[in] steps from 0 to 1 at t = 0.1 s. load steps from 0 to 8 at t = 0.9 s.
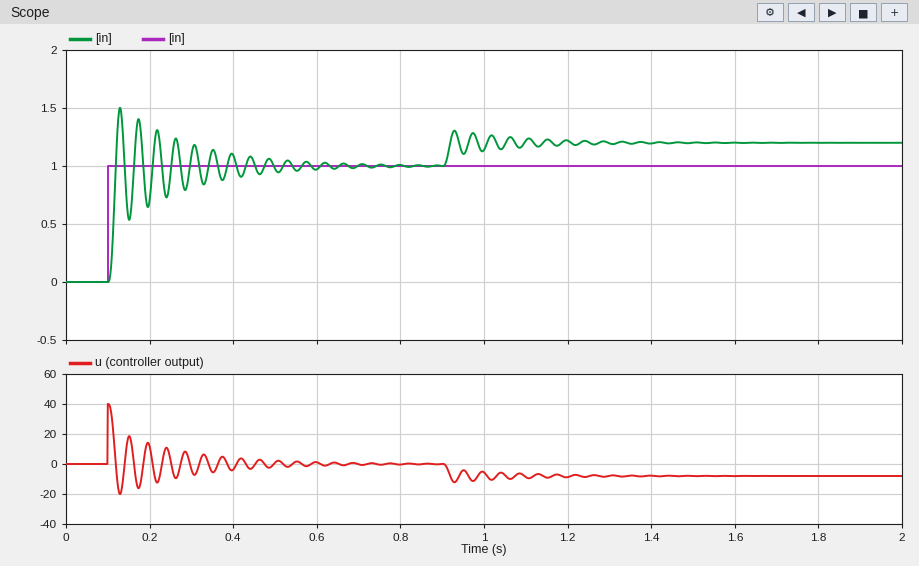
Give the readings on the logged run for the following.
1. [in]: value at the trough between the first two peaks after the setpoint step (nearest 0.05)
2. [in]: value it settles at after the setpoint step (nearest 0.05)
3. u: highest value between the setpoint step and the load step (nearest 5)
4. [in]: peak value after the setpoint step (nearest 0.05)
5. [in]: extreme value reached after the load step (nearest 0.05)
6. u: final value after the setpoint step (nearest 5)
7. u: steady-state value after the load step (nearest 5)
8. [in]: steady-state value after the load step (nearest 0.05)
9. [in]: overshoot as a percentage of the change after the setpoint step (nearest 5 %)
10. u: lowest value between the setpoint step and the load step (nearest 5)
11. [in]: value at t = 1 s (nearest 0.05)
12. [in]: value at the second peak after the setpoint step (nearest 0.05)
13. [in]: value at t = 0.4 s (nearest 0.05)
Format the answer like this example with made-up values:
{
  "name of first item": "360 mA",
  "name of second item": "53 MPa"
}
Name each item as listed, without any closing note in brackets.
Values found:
{
  "[in]: value at the trough between the first two peaks after the setpoint step": "0.55",
  "[in]: value it settles at after the setpoint step": "1.00",
  "u: highest value between the setpoint step and the load step": "40",
  "[in]: peak value after the setpoint step": "1.50",
  "[in]: extreme value reached after the load step": "1.30",
  "u: final value after the setpoint step": "0",
  "u: steady-state value after the load step": "-10",
  "[in]: steady-state value after the load step": "1.20",
  "[in]: overshoot as a percentage of the change after the setpoint step": "50 %",
  "u: lowest value between the setpoint step and the load step": "-20",
  "[in]: value at t = 1 s": "1.15",
  "[in]: value at the second peak after the setpoint step": "1.40",
  "[in]: value at t = 0.4 s": "1.10"
}
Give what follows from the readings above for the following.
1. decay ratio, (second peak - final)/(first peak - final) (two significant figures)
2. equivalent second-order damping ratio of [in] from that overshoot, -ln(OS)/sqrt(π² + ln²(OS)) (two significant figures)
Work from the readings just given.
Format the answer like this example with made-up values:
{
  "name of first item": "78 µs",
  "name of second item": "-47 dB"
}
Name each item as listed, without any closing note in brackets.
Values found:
{
  "decay ratio, (second peak - final)/(first peak - final)": "0.80",
  "equivalent second-order damping ratio of [in] from that overshoot, -ln(OS)/sqrt(π² + ln²(OS))": "0.22"
}
